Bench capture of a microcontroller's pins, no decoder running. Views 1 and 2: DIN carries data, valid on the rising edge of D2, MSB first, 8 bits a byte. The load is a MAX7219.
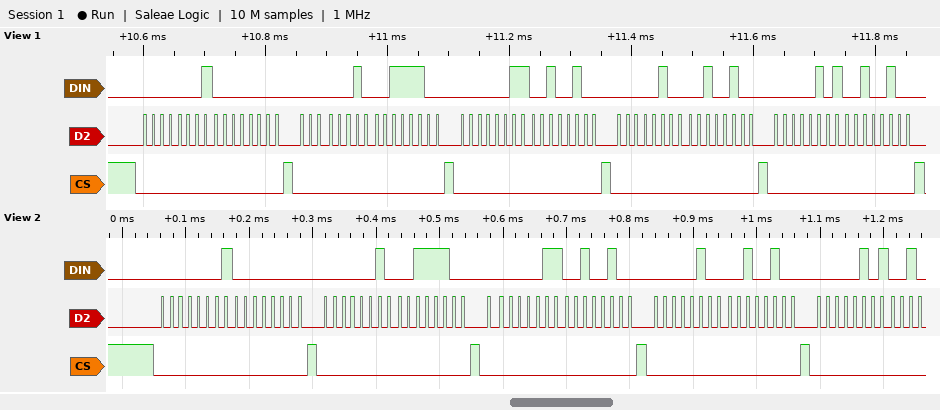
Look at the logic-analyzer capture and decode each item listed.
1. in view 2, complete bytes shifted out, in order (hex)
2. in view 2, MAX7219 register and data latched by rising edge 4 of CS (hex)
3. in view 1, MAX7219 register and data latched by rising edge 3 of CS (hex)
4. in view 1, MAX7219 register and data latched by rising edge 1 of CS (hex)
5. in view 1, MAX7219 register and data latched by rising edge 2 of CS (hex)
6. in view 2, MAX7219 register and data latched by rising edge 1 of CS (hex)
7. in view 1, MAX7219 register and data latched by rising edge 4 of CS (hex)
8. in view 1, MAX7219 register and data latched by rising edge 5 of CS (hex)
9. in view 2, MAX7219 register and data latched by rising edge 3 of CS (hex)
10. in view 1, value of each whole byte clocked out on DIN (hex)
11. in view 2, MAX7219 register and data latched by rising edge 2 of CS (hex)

0x01 0x00 0x02 0x3C 0x03 0x24 0x04 0x24 0x05
register 0x4, data 0x24
register 0x3, data 0x24
register 0x1, data 0x00
register 0x2, data 0x3C
register 0x1, data 0x00
register 0x4, data 0x24
register 0x5, data 0x24
register 0x3, data 0x24
01 00 02 3C 03 24 04 24 05 24
register 0x2, data 0x3C
